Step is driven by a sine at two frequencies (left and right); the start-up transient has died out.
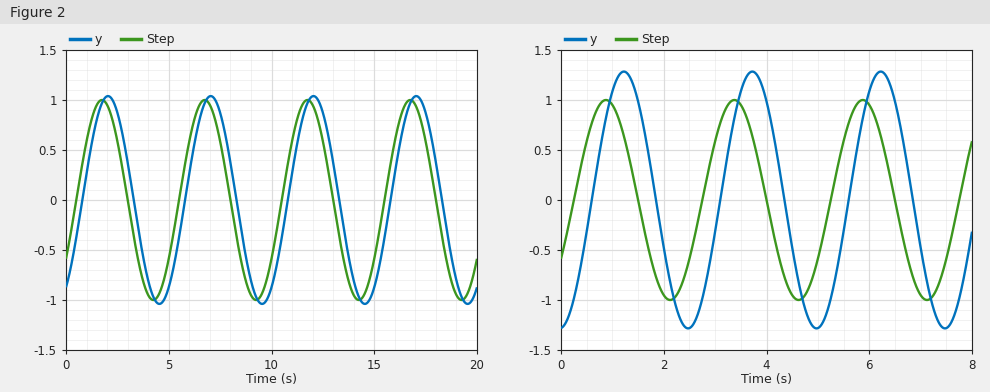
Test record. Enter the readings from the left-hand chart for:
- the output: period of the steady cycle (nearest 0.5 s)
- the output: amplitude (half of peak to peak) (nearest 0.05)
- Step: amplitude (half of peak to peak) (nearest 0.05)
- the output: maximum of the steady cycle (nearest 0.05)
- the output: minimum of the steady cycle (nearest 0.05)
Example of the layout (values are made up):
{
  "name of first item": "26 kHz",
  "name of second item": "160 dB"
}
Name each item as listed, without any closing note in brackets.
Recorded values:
{
  "the output: period of the steady cycle": "5.0 s",
  "the output: amplitude (half of peak to peak)": "1.05",
  "Step: amplitude (half of peak to peak)": "1.00",
  "the output: maximum of the steady cycle": "1.05",
  "the output: minimum of the steady cycle": "-1.05"
}
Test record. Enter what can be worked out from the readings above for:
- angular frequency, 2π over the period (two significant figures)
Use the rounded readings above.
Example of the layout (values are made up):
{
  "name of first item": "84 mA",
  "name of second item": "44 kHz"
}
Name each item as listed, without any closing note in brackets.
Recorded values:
{
  "angular frequency, 2π over the period": "1.3 rad/s"
}
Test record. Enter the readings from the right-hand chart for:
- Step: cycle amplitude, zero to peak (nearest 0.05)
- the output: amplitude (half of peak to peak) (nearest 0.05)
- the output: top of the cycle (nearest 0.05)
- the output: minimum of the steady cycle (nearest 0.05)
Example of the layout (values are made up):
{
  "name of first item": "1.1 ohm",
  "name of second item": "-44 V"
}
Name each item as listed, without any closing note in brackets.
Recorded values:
{
  "Step: cycle amplitude, zero to peak": "1.00",
  "the output: amplitude (half of peak to peak)": "1.30",
  "the output: top of the cycle": "1.30",
  "the output: minimum of the steady cycle": "-1.30"
}
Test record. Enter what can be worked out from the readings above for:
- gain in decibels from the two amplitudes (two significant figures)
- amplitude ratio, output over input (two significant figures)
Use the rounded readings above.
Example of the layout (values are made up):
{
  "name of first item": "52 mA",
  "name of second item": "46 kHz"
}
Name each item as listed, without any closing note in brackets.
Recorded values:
{
  "gain in decibels from the two amplitudes": "2.3 dB",
  "amplitude ratio, output over input": "1.3"
}
